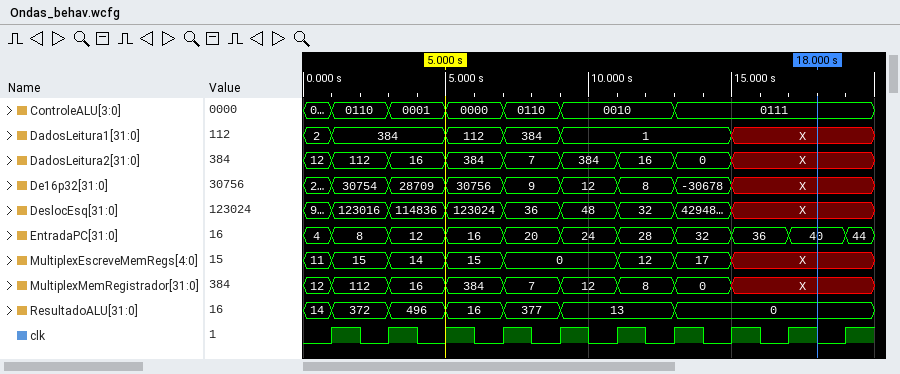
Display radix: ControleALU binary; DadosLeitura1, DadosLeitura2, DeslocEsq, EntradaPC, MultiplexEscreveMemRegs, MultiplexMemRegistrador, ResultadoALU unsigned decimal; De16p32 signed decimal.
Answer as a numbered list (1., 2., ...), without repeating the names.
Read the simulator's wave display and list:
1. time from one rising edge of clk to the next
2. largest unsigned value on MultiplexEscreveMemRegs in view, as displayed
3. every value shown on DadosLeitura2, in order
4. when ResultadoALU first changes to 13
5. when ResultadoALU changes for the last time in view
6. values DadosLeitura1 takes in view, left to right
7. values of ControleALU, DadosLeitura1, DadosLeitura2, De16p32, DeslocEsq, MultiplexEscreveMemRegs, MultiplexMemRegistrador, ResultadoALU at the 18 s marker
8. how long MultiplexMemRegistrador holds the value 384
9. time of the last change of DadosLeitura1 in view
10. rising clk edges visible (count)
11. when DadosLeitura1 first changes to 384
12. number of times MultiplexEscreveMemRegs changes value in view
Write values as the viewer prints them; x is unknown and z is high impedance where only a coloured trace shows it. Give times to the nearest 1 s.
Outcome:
1. 2 s
2. 17
3. 12, 112, 16, 384, 7, 384, 16, 0, X
4. 9 s
5. 13 s
6. 2, 384, 112, 384, 1, X
7. ControleALU=0111, DadosLeitura1=X, DadosLeitura2=X, De16p32=X, DeslocEsq=X, MultiplexEscreveMemRegs=X, MultiplexMemRegistrador=X, ResultadoALU=0
8. 2 s
9. 15 s
10. 10
11. 1 s
12. 7
